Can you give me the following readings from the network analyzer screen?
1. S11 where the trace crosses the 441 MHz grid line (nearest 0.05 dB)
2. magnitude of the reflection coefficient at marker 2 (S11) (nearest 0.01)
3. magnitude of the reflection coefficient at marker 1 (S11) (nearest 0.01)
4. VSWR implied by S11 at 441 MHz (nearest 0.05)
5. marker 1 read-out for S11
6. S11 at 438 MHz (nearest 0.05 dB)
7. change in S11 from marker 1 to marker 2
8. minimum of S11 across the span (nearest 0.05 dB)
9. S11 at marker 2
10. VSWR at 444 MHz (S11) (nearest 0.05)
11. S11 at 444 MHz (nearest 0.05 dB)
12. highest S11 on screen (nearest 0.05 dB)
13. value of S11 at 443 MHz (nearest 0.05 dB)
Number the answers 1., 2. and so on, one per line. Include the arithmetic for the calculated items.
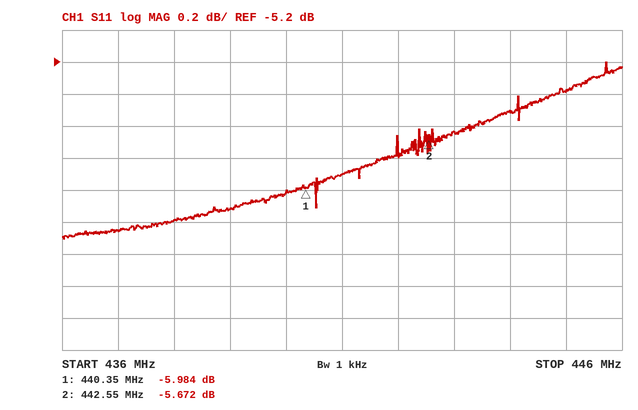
1. -5.90 dB
2. 10^(-5.672/20) ≈ 0.52
3. 10^(-5.984/20) ≈ 0.50
4. |Γ| = 10^(-5.9/20) = 0.5070; VSWR = (1 + 0.5070)/(1 − 0.5070) ≈ 3.06, so 3.05 to the nearest 0.05
5. -5.984 dB
6. -6.20 dB
7. -5.672 − (-5.984) = 0.312 dB
8. -6.30 dB
9. -5.672 dB
10. |Γ| = 10^(-5.5/20) = 0.5309; VSWR = (1 + 0.5309)/(1 − 0.5309) ≈ 3.26, so 3.25 to the nearest 0.05
11. -5.50 dB
12. -5.20 dB
13. -5.65 dB
